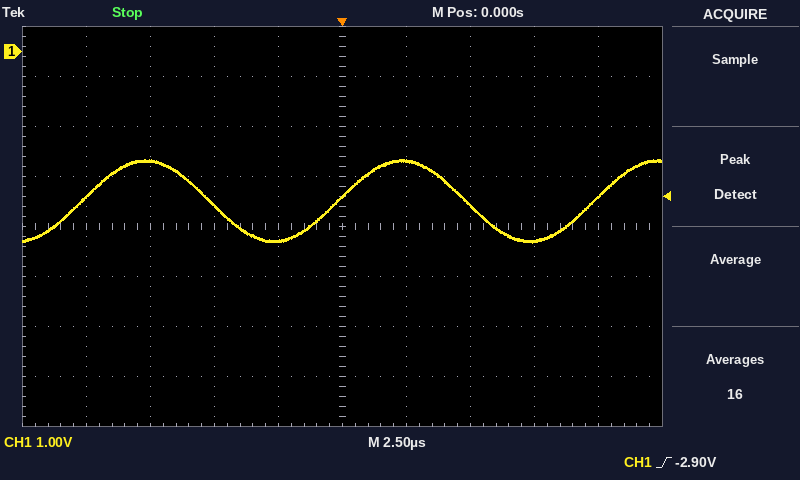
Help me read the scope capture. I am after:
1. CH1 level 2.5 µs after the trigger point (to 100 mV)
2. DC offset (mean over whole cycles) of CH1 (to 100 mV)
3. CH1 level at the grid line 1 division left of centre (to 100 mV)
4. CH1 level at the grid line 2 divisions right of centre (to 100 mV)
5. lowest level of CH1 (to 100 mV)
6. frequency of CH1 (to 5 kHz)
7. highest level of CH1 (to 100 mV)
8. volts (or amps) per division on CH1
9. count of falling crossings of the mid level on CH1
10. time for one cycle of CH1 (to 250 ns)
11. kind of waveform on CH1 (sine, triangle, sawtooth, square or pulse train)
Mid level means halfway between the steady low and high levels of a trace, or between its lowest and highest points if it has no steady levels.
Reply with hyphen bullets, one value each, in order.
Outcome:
- -2.2 V
- -3.0 V
- -3.8 V
- -3.1 V
- -3.8 V
- 100 kHz
- -2.2 V
- 1 V
- 2
- 10.00 µs
- sine
